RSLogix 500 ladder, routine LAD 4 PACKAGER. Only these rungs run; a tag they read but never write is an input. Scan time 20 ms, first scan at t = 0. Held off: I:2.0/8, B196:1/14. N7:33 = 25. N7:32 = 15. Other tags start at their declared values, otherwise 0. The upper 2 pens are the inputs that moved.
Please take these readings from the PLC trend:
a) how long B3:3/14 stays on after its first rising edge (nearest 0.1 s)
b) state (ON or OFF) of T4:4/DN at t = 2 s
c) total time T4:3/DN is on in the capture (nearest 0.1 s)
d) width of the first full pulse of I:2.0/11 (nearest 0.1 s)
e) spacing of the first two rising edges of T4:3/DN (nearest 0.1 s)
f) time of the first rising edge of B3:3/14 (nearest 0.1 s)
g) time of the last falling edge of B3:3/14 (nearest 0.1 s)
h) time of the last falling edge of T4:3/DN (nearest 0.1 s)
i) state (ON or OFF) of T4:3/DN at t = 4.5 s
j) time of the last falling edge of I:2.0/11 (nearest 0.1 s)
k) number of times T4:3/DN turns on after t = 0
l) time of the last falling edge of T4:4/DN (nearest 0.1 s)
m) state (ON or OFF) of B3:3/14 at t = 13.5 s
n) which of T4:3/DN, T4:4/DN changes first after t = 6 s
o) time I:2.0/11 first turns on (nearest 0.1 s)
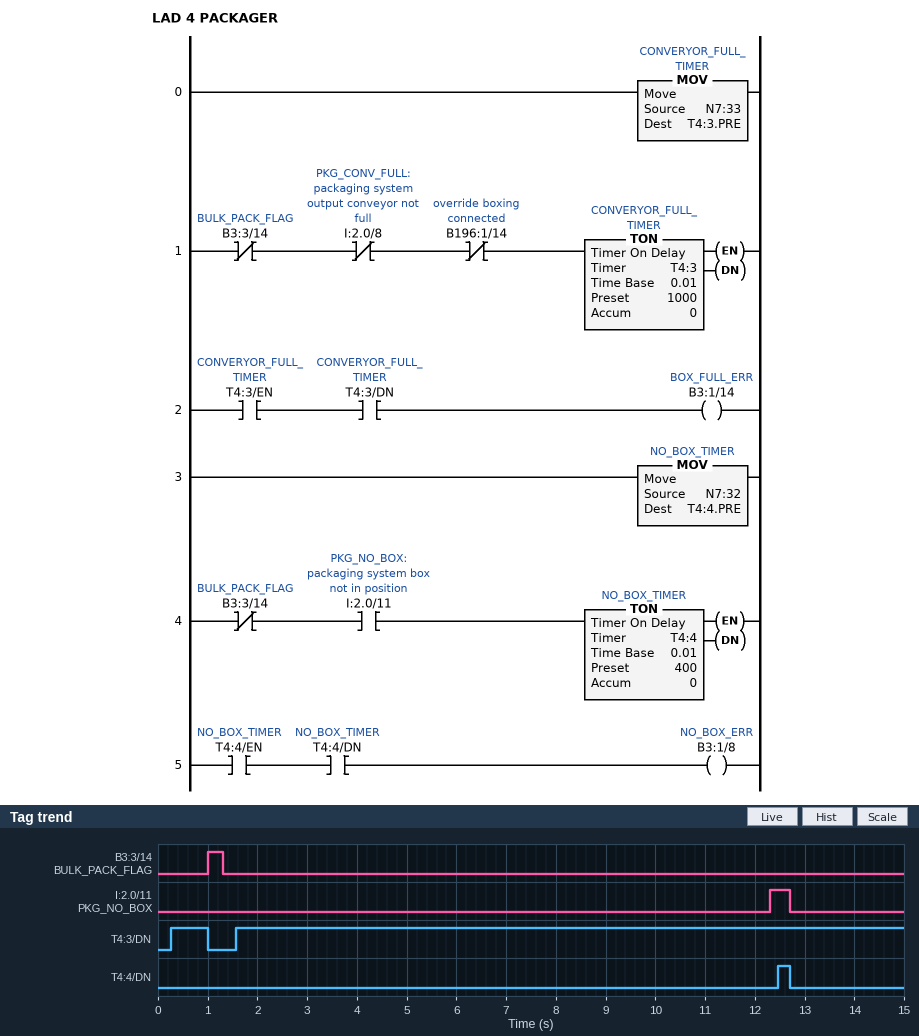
0.3 s
OFF
14.2 s
0.4 s
1.3 s
1.0 s
1.3 s
1.0 s
ON
12.7 s
2
12.7 s
OFF
T4:4/DN
12.3 s
